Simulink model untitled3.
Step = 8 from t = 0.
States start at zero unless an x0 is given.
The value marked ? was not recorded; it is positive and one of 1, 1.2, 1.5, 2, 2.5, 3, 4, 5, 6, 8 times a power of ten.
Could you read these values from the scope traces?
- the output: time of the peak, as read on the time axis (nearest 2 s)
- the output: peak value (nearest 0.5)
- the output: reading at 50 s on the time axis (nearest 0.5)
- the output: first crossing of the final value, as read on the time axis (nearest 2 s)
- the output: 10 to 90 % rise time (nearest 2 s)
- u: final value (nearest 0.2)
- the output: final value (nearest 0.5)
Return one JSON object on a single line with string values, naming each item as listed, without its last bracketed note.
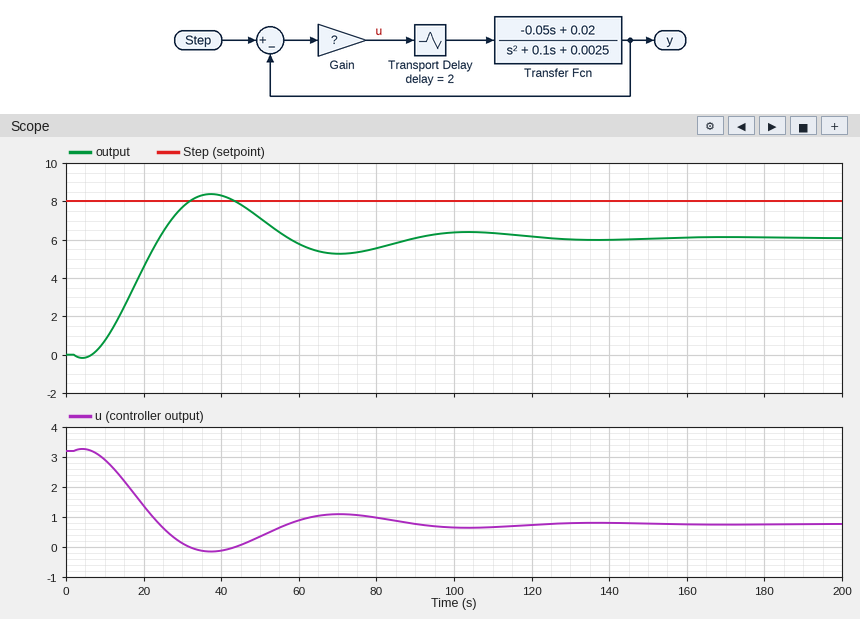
{"the output: time of the peak, as read on the time axis": "38 s", "the output: peak value": "8.5", "the output: reading at 50 s on the time axis": "7.0", "the output: first crossing of the final value, as read on the time axis": "24 s", "the output: 10 to 90 % rise time": "12 s", "u: final value": "0.8", "the output: final value": "6.0"}
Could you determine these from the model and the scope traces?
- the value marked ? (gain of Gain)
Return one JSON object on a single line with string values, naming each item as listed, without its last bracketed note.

{"the value marked ?": "0.4"}
